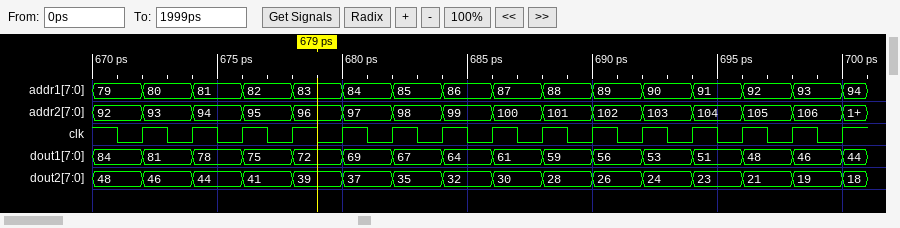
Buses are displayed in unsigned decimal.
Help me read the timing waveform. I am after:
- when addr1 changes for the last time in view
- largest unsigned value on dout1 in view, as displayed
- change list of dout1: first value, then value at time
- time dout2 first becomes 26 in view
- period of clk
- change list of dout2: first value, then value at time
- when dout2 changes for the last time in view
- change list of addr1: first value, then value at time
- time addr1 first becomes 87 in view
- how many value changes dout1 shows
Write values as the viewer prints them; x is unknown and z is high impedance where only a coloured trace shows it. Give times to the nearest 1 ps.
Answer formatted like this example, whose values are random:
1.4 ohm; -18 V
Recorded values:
700 ps; 84; 84, 81 at 672 ps, 78 at 674 ps, 75 at 676 ps, 72 at 678 ps, 69 at 680 ps, 67 at 682 ps, 64 at 684 ps, 61 at 686 ps, 59 at 688 ps, 56 at 690 ps, 53 at 692 ps, 51 at 694 ps, 48 at 696 ps, 46 at 698 ps, 44 at 700 ps; 690 ps; 2 ps; 48, 46 at 672 ps, 44 at 674 ps, 41 at 676 ps, 39 at 678 ps, 37 at 680 ps, 35 at 682 ps, 32 at 684 ps, 30 at 686 ps, 28 at 688 ps, 26 at 690 ps, 24 at 692 ps, 23 at 694 ps, 21 at 696 ps, 19 at 698 ps, 18 at 700 ps; 700 ps; 79, 80 at 672 ps, 81 at 674 ps, 82 at 676 ps, 83 at 678 ps, 84 at 680 ps, 85 at 682 ps, 86 at 684 ps, 87 at 686 ps, 88 at 688 ps, 89 at 690 ps, 90 at 692 ps, 91 at 694 ps, 92 at 696 ps, 93 at 698 ps, 94 at 700 ps; 686 ps; 15
